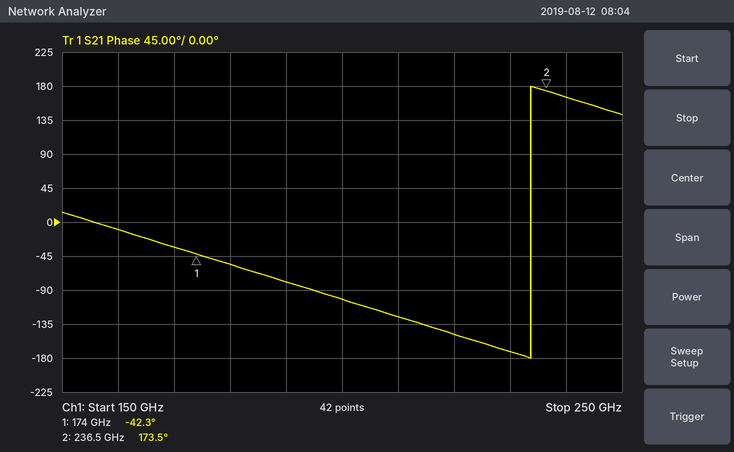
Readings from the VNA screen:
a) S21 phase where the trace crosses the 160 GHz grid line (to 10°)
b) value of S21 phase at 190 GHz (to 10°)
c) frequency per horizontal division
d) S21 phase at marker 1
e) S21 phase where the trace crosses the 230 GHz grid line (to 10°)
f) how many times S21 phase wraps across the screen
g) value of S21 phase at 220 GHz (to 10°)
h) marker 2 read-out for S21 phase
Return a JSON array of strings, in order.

["-10°", "-80°", "10 GHz", "-42.3°", "-170°", "1", "-150°", "173.5°"]
